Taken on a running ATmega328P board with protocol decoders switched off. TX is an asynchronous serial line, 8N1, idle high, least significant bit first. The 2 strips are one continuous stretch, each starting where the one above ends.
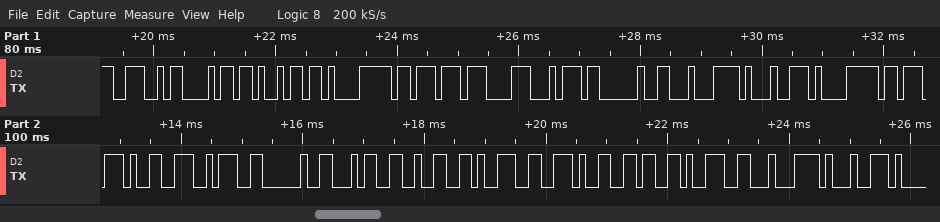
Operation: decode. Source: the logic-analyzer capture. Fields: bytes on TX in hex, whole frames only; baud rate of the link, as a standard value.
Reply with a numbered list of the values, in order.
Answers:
1. 4E 68 69 E1 BB 87 74 20 C4 91 E1 BB 99 3A 20 34 32 39 2E 36 39 C4 91
2. 9600 baud
